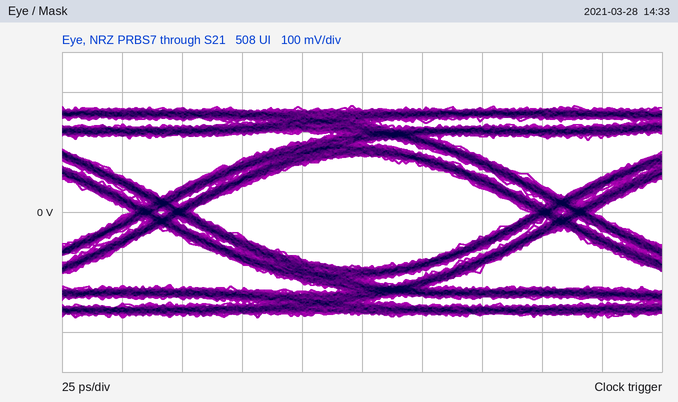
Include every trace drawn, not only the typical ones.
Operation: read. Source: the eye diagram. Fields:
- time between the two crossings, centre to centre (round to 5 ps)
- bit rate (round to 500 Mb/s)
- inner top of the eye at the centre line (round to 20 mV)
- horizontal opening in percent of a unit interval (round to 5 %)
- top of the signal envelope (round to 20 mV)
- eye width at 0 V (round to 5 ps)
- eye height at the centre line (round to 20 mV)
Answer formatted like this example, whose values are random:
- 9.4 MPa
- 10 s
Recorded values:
- 165 ps
- 6.0 Gb/s
- 140 mV
- 85 %
- 260 mV
- 140 ps
- 280 mV
